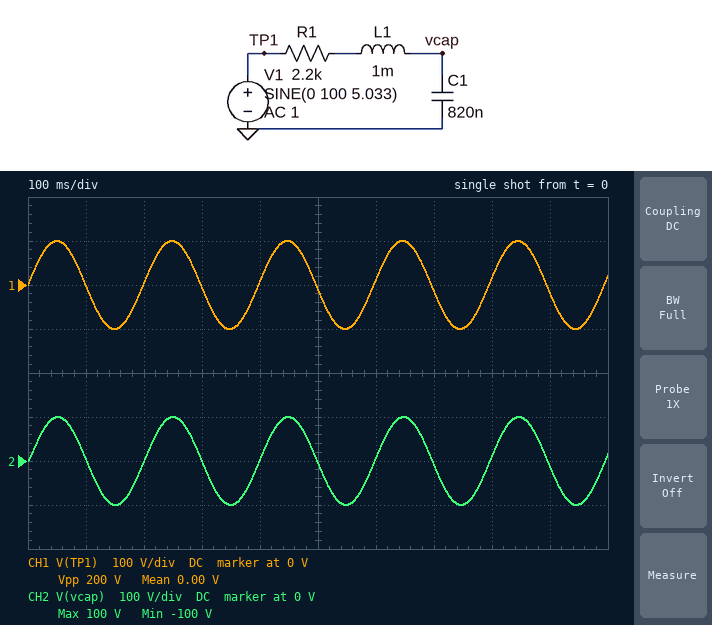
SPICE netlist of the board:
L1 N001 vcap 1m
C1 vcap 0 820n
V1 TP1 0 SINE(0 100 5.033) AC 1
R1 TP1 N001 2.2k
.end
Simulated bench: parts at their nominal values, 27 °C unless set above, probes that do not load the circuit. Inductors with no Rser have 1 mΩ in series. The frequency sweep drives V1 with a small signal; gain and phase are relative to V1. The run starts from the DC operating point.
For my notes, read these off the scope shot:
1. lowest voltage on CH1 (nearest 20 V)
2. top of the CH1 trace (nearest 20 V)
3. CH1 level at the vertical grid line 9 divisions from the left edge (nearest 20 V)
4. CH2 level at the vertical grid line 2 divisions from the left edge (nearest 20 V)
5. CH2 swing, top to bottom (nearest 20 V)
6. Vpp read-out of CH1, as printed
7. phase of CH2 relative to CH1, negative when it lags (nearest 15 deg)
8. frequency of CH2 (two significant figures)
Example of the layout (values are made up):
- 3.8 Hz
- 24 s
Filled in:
- -100 V
- 100 V
- -20 V
- 0 V
- 200 V
- 200 V
- 0 deg
- 5.0 Hz
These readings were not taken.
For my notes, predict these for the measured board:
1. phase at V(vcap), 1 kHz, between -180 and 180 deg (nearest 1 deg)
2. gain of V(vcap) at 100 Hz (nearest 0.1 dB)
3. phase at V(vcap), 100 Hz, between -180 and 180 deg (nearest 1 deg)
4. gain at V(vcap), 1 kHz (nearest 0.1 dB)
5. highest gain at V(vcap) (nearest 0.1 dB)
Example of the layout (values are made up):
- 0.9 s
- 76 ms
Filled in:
- -85 deg
- -3.6 dB
- -49 deg
- -21.1 dB
- 0 dB
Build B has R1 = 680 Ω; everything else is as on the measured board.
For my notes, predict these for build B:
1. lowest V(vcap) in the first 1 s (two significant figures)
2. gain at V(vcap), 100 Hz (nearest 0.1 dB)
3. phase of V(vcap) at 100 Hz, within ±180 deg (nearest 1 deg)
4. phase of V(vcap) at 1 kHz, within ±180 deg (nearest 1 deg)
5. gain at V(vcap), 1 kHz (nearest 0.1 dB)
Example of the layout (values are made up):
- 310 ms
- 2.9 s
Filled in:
- -100 V
- -0.5 dB
- -19 deg
- -75 deg
- -11.2 dB
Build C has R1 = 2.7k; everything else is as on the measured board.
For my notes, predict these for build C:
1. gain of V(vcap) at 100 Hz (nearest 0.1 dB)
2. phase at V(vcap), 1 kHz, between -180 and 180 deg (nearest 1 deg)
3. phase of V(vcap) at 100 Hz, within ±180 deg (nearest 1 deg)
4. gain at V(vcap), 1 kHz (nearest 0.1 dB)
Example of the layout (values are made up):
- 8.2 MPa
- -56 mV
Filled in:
- -4.7 dB
- -86 deg
- -54 deg
- -22.9 dB
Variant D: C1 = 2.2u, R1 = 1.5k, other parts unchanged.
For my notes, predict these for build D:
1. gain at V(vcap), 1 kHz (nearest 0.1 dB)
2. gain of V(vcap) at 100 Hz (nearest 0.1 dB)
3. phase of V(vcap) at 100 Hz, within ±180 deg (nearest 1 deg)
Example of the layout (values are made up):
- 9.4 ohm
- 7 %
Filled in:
- -26.3 dB
- -7.2 dB
- -64 deg
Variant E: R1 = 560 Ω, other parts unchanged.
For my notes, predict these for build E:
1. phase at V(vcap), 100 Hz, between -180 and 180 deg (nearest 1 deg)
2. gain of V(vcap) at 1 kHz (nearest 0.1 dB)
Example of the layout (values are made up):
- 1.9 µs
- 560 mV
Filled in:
- -16 deg
- -9.7 dB
